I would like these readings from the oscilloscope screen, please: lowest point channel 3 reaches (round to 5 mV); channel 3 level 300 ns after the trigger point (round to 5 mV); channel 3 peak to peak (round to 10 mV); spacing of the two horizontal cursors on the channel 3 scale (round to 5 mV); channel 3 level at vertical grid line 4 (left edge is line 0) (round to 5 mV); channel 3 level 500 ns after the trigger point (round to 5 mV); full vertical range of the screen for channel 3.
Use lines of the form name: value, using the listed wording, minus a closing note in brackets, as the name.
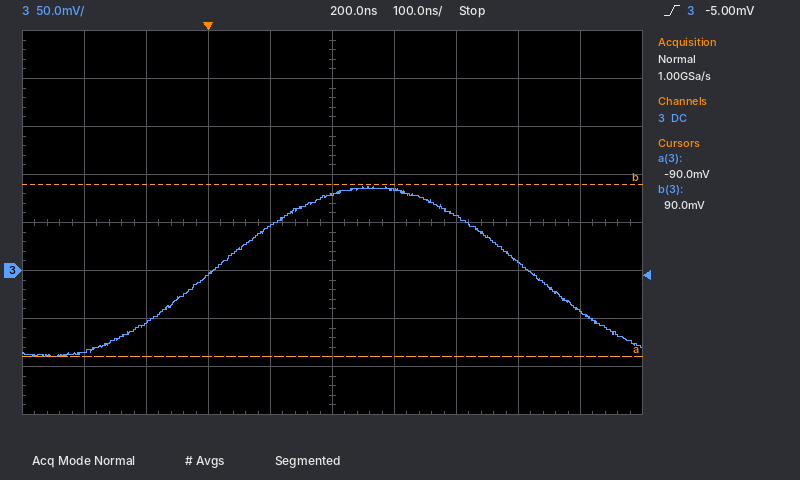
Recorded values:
lowest point channel 3 reaches: -90 mV
channel 3 level 300 ns after the trigger point: 85 mV
channel 3 peak to peak: 180 mV
spacing of the two horizontal cursors on the channel 3 scale: 180 mV
channel 3 level at vertical grid line 4 (left edge is line 0): 45 mV
channel 3 level 500 ns after the trigger point: 10 mV
full vertical range of the screen for channel 3: 400 mV
